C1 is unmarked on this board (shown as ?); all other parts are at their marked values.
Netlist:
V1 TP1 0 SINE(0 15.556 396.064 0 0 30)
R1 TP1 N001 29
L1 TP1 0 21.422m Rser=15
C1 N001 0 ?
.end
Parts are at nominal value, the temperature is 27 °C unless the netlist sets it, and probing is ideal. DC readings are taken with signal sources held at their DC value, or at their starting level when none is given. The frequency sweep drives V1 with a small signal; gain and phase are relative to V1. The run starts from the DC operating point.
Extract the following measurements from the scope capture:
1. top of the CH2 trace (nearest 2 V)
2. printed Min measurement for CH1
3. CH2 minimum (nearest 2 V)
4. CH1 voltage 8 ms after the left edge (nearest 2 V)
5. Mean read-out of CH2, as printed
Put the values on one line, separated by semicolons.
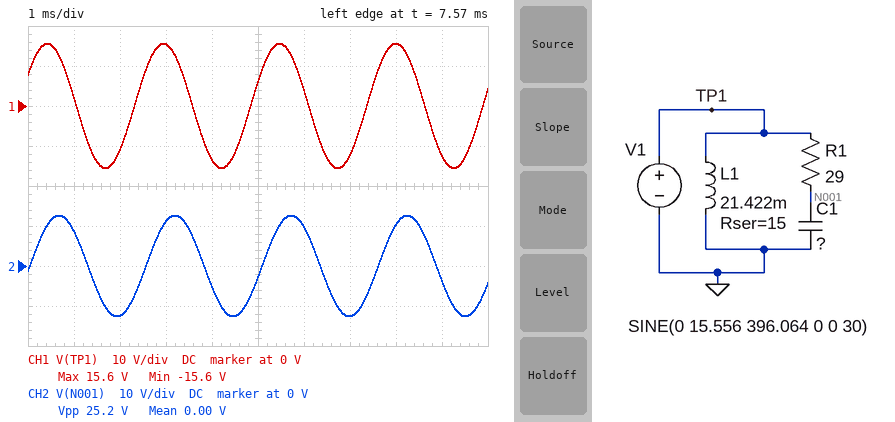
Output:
12 V; -15.6 V; -12 V; 16 V; 0.00 V
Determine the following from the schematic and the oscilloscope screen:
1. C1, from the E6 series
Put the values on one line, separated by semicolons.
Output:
10 µF
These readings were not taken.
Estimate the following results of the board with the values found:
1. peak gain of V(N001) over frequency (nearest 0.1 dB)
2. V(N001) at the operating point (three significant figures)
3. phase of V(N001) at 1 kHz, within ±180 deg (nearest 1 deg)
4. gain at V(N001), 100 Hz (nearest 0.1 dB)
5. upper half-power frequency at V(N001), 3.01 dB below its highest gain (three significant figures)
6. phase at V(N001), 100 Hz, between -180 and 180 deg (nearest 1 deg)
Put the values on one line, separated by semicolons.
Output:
0 dB; 7.78 V; -61 deg; -0.1 dB; 549 Hz; -10 deg
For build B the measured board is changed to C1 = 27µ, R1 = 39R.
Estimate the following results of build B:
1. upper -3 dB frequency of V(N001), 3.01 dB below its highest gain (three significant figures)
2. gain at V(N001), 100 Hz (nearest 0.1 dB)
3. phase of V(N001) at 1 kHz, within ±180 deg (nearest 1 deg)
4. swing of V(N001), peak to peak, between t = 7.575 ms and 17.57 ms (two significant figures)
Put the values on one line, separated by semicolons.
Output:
151 Hz; -1.6 dB; -81 deg; 11 V
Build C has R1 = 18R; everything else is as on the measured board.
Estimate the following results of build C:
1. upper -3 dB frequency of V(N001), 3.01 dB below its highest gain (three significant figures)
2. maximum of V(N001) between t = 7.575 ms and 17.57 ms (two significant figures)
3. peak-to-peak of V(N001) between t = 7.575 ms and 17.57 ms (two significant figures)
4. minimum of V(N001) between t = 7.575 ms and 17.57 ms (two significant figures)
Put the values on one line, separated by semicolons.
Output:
884 Hz; 14 V; 28 V; -14 V
